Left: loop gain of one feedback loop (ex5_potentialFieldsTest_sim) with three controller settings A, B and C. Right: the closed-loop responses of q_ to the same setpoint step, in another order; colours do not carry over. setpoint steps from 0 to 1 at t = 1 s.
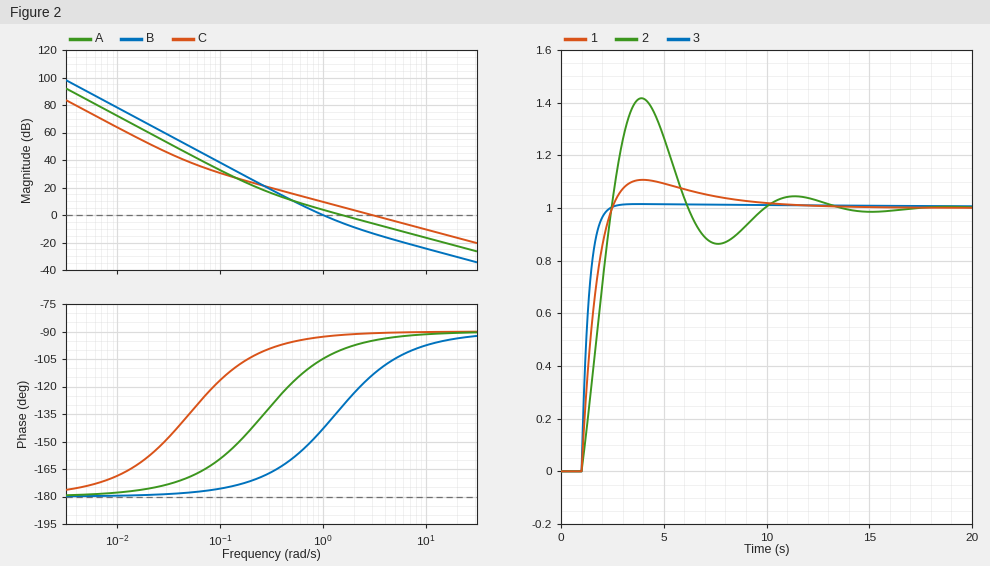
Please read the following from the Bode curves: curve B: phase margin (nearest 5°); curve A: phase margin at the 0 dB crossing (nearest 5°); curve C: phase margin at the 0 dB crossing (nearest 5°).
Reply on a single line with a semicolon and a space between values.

35°; 80°; 90°
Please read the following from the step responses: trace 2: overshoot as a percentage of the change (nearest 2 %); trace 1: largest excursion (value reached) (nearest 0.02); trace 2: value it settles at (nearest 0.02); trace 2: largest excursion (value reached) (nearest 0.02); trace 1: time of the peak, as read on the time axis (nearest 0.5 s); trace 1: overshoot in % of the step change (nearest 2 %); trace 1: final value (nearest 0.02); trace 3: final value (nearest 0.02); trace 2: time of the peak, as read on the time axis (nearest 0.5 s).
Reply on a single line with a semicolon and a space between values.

42 %; 1.10; 1.00; 1.42; 4.0 s; 10 %; 1.00; 1.00; 4.0 s
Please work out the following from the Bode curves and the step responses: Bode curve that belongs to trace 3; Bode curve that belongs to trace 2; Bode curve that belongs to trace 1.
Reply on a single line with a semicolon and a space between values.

C; B; A
